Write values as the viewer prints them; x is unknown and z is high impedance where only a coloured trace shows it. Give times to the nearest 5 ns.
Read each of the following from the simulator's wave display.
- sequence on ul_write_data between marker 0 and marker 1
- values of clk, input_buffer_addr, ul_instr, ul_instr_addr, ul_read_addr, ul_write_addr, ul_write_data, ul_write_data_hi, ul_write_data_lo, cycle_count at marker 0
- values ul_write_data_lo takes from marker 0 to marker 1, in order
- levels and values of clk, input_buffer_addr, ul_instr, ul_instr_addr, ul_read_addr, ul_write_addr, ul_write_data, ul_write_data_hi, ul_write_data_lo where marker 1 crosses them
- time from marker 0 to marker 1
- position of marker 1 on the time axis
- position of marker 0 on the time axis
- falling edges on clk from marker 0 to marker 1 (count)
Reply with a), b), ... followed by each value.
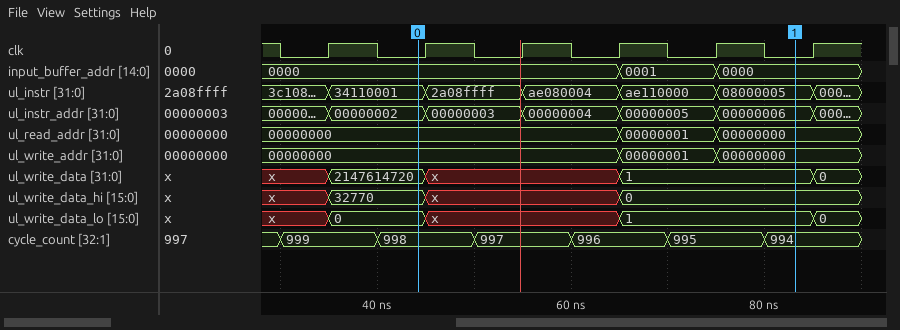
a) 2147614720, x, 1
b) clk=0, input_buffer_addr=0000, ul_instr=34110001, ul_instr_addr=00000002, ul_read_addr=00000000, ul_write_addr=00000000, ul_write_data=2147614720, ul_write_data_hi=32770, ul_write_data_lo=0, cycle_count=998
c) 0, x, 1
d) clk=0, input_buffer_addr=0000, ul_instr=08000005, ul_instr_addr=00000006, ul_read_addr=00000000, ul_write_addr=00000000, ul_write_data=1, ul_write_data_hi=0, ul_write_data_lo=1
e) 40 ns
f) 85 ns
g) 45 ns
h) 4
